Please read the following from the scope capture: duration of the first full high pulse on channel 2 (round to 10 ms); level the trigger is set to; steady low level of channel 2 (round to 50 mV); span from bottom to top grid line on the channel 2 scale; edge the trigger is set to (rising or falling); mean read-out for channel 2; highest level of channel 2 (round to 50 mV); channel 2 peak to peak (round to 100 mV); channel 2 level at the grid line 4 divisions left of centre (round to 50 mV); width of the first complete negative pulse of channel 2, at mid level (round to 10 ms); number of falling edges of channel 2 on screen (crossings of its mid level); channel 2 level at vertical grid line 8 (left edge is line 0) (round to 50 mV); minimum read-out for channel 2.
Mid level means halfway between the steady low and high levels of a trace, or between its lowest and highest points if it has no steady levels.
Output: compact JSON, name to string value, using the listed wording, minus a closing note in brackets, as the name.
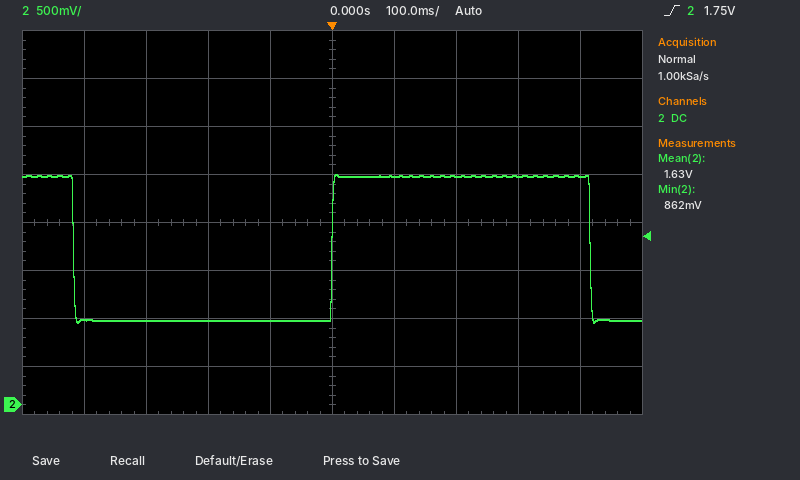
{"duration of the first full high pulse on channel 2": "420 ms", "level the trigger is set to": "1.75 V", "steady low level of channel 2": "900 mV", "span from bottom to top grid line on the channel 2 scale": "4 V", "edge the trigger is set to": "rising", "mean read-out for channel 2": "1.63 V", "highest level of channel 2": "2.40 V", "channel 2 peak to peak": "1.50 V", "channel 2 level at the grid line 4 divisions left of centre": "900 mV", "width of the first complete negative pulse of channel 2, at mid level": "420 ms", "number of falling edges of channel 2 on screen": "2", "channel 2 level at vertical grid line 8 (left edge is line 0)": "2.40 V", "minimum read-out for channel 2": "862 mV"}
